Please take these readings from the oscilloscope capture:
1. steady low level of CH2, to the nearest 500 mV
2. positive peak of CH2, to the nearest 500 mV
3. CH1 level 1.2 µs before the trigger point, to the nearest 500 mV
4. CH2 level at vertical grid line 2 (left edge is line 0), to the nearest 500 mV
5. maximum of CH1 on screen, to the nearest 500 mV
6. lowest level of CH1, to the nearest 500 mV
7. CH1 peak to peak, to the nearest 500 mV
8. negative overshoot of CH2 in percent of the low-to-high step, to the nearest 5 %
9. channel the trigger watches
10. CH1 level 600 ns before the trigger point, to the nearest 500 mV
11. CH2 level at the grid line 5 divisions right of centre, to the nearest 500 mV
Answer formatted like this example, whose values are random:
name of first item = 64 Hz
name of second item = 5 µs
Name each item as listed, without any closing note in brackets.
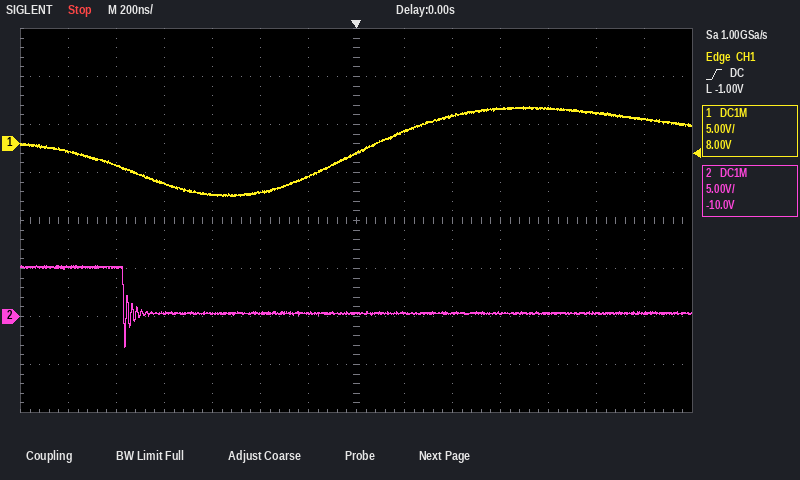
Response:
steady low level of CH2, to the nearest 500 mV = 500 mV
positive peak of CH2, to the nearest 500 mV = 5.5 V
CH1 level 1.2 µs before the trigger point, to the nearest 500 mV = -1.0 V
CH2 level at vertical grid line 2 (left edge is line 0), to the nearest 500 mV = 5.0 V
maximum of CH1 on screen, to the nearest 500 mV = 4.0 V
lowest level of CH1, to the nearest 500 mV = -5.5 V
CH1 peak to peak, to the nearest 500 mV = 9.5 V
negative overshoot of CH2 in percent of the low-to-high step, to the nearest 5 % = 75 %
channel the trigger watches = CH1
CH1 level 600 ns before the trigger point, to the nearest 500 mV = -5.5 V
CH2 level at the grid line 5 divisions right of centre, to the nearest 500 mV = 500 mV
